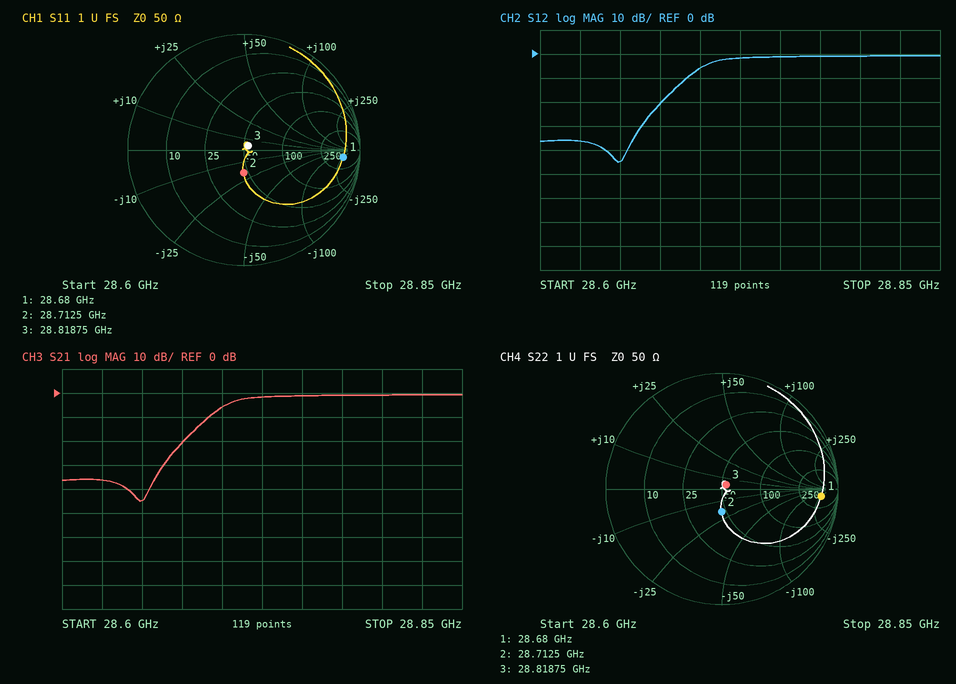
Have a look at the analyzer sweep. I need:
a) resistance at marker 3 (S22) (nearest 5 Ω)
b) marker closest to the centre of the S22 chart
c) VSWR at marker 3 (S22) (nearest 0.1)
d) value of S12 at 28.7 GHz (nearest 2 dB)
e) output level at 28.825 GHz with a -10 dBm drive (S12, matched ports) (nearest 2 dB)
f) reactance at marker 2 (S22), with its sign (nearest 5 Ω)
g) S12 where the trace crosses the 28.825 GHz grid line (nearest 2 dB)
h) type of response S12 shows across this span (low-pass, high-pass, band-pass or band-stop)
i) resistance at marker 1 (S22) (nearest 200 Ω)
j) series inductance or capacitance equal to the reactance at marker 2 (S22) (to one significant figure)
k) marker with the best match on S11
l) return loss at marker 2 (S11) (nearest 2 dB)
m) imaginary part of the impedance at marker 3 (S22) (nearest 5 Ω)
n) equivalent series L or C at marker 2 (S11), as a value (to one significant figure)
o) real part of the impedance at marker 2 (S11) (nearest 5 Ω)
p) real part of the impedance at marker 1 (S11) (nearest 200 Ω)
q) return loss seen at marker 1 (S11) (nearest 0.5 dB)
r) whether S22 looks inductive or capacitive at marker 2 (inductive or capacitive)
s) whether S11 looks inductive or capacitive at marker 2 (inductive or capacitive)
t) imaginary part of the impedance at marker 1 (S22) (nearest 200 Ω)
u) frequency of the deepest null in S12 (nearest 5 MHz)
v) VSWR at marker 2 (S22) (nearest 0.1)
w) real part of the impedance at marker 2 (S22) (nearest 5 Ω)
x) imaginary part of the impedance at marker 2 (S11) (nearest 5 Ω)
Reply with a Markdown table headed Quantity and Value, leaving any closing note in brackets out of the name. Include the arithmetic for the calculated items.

| Quantity | Value |
|---|---|
| resistance at marker 3 (S22) | 55 Ω |
| marker closest to the centre of the S22 chart | marker 3 |
| VSWR at marker 3 (S22) | 1.1 |
| value of S12 at 28.7 GHz | -6 dB |
| output level at 28.825 GHz with a -10 dBm drive (S12, matched ports) | -10 dBm + (0 dB) = -10 dBm |
| reactance at marker 2 (S22), with its sign | -20 Ω |
| S12 where the trace crosses the 28.825 GHz grid line | 0 dB |
| type of response S12 shows across this span | high-pass |
| resistance at marker 1 (S22) | 600 Ω |
| series inductance or capacitance equal to the reactance at marker 2 (S22) | C = 1/(2π × 28.7125 GHz × 20 Ω) ≈ 277 fF, so 300 fF to one significant figure |
| marker with the best match on S11 | marker 3 |
| return loss at marker 2 (S11) | 14 dB |
| imaginary part of the impedance at marker 3 (S22) | +5 Ω |
| equivalent series L or C at marker 2 (S11), as a value | C = 1/(2π × 28.7125 GHz × 20 Ω) ≈ 277 fF, so 300 fF to one significant figure |
| real part of the impedance at marker 2 (S11) | 45 Ω |
| real part of the impedance at marker 1 (S11) | 600 Ω |
| return loss seen at marker 1 (S11) | 1.5 dB |
| whether S22 looks inductive or capacitive at marker 2 | capacitive |
| whether S11 looks inductive or capacitive at marker 2 | capacitive |
| imaginary part of the impedance at marker 1 (S22) | -200 Ω |
| frequency of the deepest null in S12 | 28.650 GHz |
| VSWR at marker 2 (S22) | 1.5 |
| real part of the impedance at marker 2 (S22) | 45 Ω |
| imaginary part of the impedance at marker 2 (S11) | -20 Ω |
